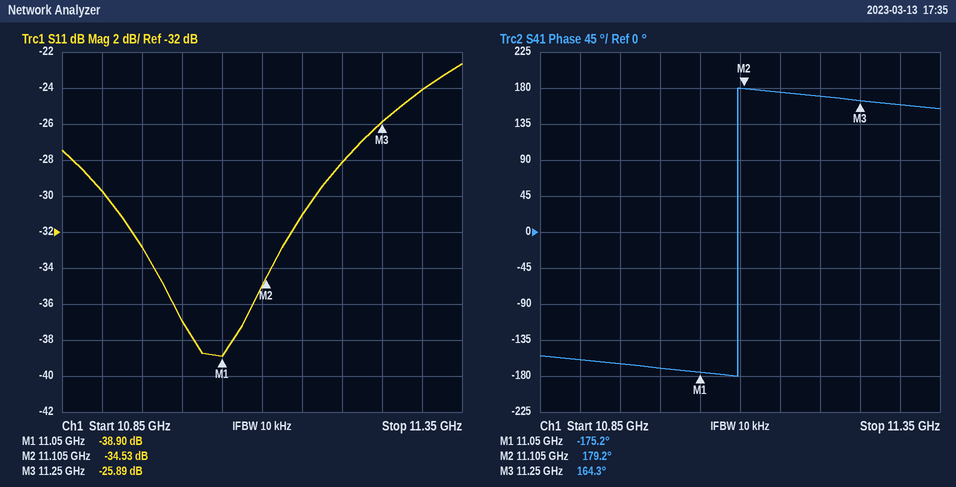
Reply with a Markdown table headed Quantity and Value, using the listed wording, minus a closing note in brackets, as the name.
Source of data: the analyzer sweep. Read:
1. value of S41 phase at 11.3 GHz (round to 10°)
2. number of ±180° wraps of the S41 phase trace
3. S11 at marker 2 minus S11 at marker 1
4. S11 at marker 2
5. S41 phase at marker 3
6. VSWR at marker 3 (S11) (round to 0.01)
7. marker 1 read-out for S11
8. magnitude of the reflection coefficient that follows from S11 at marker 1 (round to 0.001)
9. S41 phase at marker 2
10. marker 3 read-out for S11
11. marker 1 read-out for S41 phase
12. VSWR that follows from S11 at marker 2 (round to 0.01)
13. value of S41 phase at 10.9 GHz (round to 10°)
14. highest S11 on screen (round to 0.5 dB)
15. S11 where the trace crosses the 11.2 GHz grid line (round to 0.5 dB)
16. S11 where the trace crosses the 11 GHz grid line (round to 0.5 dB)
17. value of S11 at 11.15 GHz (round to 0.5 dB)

| Quantity | Value |
|---|---|
| value of S41 phase at 11.3 GHz | 160° |
| number of ±180° wraps of the S41 phase trace | 1 |
| S11 at marker 2 minus S11 at marker 1 | 4.37 dB |
| S11 at marker 2 | -34.53 dB |
| S41 phase at marker 3 | 164.3° |
| VSWR at marker 3 (S11) | 1.11 |
| marker 1 read-out for S11 | -38.90 dB |
| magnitude of the reflection coefficient that follows from S11 at marker 1 | 0.011 |
| S41 phase at marker 2 | 179.2° |
| marker 3 read-out for S11 | -25.89 dB |
| marker 1 read-out for S41 phase | -175.2° |
| VSWR that follows from S11 at marker 2 | 1.04 |
| value of S41 phase at 10.9 GHz | -160° |
| highest S11 on screen | -22.5 dB |
| S11 where the trace crosses the 11.2 GHz grid line | -28.0 dB |
| S11 where the trace crosses the 11 GHz grid line | -37.0 dB |
| value of S11 at 11.15 GHz | -31.0 dB |
